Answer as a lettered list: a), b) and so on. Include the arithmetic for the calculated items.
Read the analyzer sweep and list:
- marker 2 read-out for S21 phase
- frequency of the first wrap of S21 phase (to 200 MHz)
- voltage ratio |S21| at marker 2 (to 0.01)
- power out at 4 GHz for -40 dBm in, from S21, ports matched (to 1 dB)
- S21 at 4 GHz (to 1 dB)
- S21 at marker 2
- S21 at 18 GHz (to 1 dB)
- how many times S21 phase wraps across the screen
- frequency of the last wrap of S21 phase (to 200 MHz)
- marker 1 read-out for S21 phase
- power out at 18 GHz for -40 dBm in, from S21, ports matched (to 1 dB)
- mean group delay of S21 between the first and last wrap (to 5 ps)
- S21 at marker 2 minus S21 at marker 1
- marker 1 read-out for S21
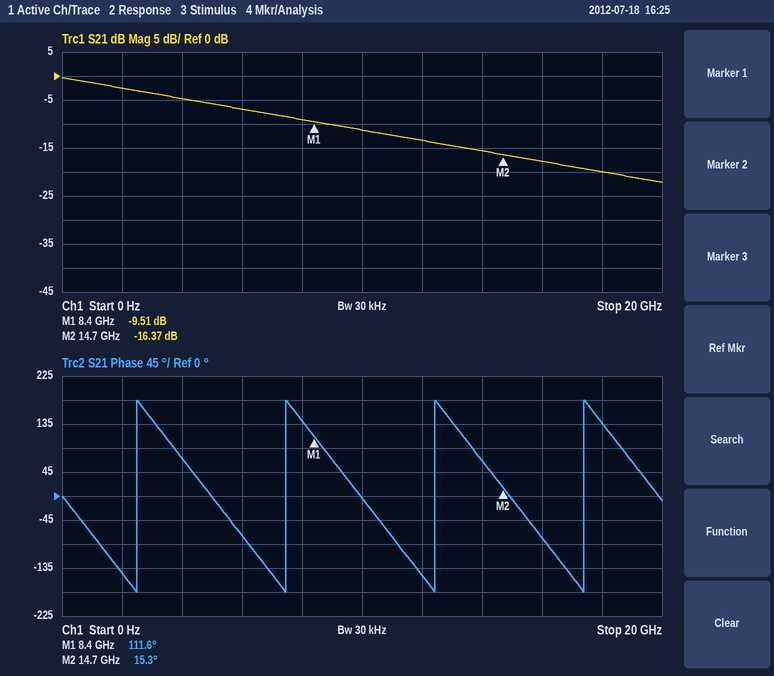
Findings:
a) 15.3°
b) 2.4 GHz
c) 10^(-16.37/20) ≈ 0.15
d) -40 dBm + (-5 dB) = -45 dBm
e) -5 dB
f) -16.37 dB
g) -20 dB
h) 4
i) 17.4 GHz
j) 111.6°
k) -40 dBm + (-20 dB) = -60 dBm
l) 3 cycles / (17.4 GHz − 2.4 GHz) ≈ 200 ps
m) -16.37 − (-9.51) = -6.86 dB
n) -9.51 dB
